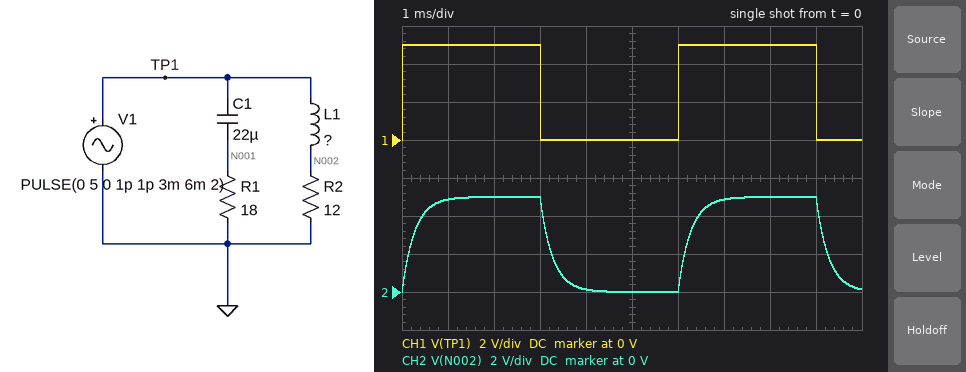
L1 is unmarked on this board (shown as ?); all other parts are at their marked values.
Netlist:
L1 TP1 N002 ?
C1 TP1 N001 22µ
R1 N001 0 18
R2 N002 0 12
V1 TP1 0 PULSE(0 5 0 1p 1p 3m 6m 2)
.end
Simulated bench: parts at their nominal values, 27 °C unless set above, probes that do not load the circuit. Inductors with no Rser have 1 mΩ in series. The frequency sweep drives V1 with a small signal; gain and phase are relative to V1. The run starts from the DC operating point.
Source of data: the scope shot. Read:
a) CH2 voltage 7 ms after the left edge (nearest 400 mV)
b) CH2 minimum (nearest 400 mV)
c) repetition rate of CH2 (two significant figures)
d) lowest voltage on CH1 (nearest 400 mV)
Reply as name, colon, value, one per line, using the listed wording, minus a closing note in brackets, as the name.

CH2 voltage 7 ms after the left edge: 4.8 V
CH2 minimum: 0 V
repetition rate of CH2: 170 Hz
lowest voltage on CH1: 0 V
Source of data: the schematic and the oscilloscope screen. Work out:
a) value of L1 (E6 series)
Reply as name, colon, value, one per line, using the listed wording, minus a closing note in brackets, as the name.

value of L1: 3.3 mH
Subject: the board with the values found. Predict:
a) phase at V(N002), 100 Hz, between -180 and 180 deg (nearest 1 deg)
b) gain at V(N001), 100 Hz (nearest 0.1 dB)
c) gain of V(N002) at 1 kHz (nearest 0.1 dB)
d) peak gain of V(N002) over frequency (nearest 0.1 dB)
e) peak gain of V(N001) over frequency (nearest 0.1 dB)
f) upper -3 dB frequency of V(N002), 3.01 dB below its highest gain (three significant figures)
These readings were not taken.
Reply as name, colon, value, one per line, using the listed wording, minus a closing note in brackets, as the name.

phase at V(N002), 100 Hz, between -180 and 180 deg: -10 deg
gain at V(N001), 100 Hz: -12.3 dB
gain of V(N002) at 1 kHz: -6.0 dB
peak gain of V(N002) over frequency: 0 dB
peak gain of V(N001) over frequency: 0 dB
upper -3 dB frequency of V(N002), 3.01 dB below its highest gain: 579 Hz
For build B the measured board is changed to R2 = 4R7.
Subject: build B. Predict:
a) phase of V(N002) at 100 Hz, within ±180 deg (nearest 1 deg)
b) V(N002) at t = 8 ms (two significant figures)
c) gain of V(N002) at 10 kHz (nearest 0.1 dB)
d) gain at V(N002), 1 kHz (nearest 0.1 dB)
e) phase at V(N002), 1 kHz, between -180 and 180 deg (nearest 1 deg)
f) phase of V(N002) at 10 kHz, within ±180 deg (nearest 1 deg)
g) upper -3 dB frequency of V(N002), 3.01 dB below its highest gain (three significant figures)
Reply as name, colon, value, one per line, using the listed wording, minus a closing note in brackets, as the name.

phase of V(N002) at 100 Hz, within ±180 deg: -24 deg
V(N002) at t = 8 ms: 4.7 V
gain of V(N002) at 10 kHz: -32.9 dB
gain at V(N002), 1 kHz: -13.1 dB
phase at V(N002), 1 kHz, between -180 and 180 deg: -77 deg
phase of V(N002) at 10 kHz, within ±180 deg: -89 deg
upper -3 dB frequency of V(N002), 3.01 dB below its highest gain: 227 Hz
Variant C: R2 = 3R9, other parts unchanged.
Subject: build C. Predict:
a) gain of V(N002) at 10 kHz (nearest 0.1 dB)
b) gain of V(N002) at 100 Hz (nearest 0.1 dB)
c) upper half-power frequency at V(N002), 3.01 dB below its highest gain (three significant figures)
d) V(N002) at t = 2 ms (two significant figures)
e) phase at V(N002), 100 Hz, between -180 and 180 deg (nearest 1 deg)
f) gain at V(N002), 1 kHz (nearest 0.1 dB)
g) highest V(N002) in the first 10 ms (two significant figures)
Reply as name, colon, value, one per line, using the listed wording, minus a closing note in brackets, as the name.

gain of V(N002) at 10 kHz: -34.5 dB
gain of V(N002) at 100 Hz: -1.1 dB
upper half-power frequency at V(N002), 3.01 dB below its highest gain: 188 Hz
V(N002) at t = 2 ms: 4.5 V
phase at V(N002), 100 Hz, between -180 and 180 deg: -28 deg
gain at V(N002), 1 kHz: -14.7 dB
highest V(N002) in the first 10 ms: 4.9 V
